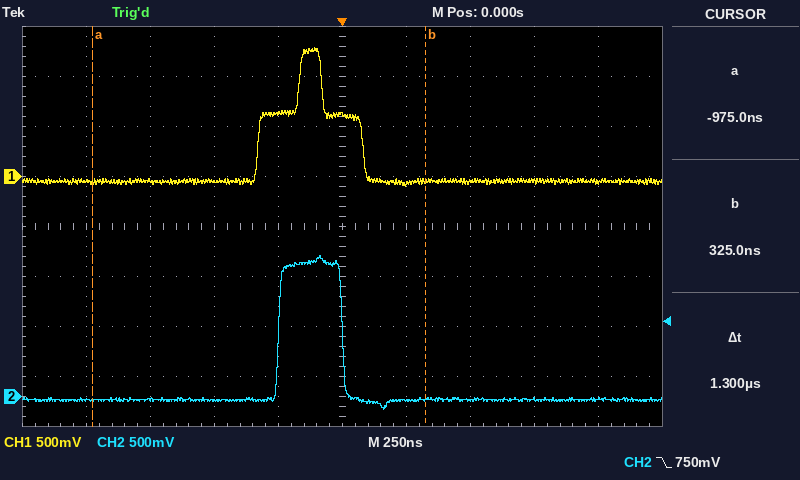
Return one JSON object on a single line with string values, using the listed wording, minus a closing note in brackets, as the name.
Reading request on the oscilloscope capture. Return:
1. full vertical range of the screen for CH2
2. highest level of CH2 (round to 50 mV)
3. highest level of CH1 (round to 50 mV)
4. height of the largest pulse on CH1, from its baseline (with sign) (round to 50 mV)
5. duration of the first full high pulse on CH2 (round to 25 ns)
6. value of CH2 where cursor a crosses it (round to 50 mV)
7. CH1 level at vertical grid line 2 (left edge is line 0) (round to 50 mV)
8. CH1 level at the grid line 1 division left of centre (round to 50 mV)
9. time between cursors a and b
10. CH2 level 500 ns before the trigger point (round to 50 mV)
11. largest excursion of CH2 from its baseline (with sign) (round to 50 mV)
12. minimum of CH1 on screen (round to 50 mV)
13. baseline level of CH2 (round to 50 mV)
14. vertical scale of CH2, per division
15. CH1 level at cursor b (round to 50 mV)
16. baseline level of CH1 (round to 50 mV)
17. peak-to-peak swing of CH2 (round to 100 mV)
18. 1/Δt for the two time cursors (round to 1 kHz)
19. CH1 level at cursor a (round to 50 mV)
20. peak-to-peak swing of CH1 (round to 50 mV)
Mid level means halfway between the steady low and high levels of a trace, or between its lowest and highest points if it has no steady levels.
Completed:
{"full vertical range of the screen for CH2": "4 V", "highest level of CH2": "1.40 V", "highest level of CH1": "1.30 V", "height of the largest pulse on CH1, from its baseline (with sign)": "+1.35 V", "duration of the first full high pulse on CH2": "250 ns", "value of CH2 where cursor a crosses it": "-50 mV", "CH1 level at vertical grid line 2 (left edge is line 0)": "-50 mV", "CH1 level at the grid line 1 division left of centre": "650 mV", "time between cursors a and b": "1.3 µs", "CH2 level 500 ns before the trigger point": "-50 mV", "largest excursion of CH2 from its baseline (with sign)": "+1.45 V", "minimum of CH1 on screen": "-100 mV", "baseline level of CH2": "-50 mV", "vertical scale of CH2, per division": "500 mV", "CH1 level at cursor b": "-50 mV", "baseline level of CH1": "-50 mV", "peak-to-peak swing of CH2": "1.50 V", "1/Δt for the two time cursors": "769 kHz", "CH1 level at cursor a": "-50 mV", "peak-to-peak swing of CH1": "1.40 V"}
